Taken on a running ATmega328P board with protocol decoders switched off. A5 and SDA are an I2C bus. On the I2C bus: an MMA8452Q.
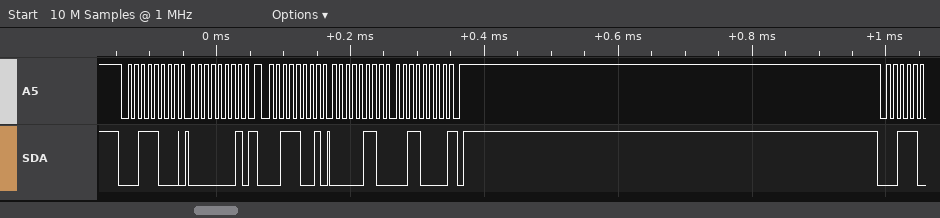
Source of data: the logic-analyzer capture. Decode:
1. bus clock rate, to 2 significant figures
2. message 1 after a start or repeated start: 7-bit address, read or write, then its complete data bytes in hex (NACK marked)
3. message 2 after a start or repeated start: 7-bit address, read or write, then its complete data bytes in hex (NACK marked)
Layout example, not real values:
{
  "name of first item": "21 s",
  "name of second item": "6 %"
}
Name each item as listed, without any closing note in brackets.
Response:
{
  "bus clock rate, to 2 significant figures": "100 kHz",
  "message 1 after a start or repeated start: 7-bit address, read or write, then its complete data bytes in hex": "0x1C write: 01",
  "message 2 after a start or repeated start: 7-bit address, read or write, then its complete data bytes in hex": "0x1C read: 06 30 NACK"
}
